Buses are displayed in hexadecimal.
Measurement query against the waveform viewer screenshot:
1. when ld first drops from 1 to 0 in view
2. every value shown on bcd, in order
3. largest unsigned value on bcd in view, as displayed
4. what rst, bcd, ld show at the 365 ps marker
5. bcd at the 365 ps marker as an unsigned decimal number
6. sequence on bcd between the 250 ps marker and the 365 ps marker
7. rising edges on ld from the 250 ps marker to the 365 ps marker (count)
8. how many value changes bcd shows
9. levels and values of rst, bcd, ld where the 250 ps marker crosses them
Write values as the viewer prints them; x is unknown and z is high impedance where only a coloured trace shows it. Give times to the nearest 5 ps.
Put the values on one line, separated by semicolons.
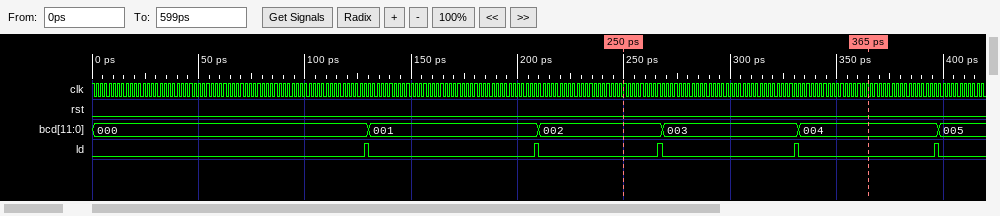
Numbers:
130 ps; 000, 001, 002, 003, 004, 005; 005; rst=0, bcd=004, ld=0; 4; 002, 003, 004; 2; 5; rst=0, bcd=002, ld=0
